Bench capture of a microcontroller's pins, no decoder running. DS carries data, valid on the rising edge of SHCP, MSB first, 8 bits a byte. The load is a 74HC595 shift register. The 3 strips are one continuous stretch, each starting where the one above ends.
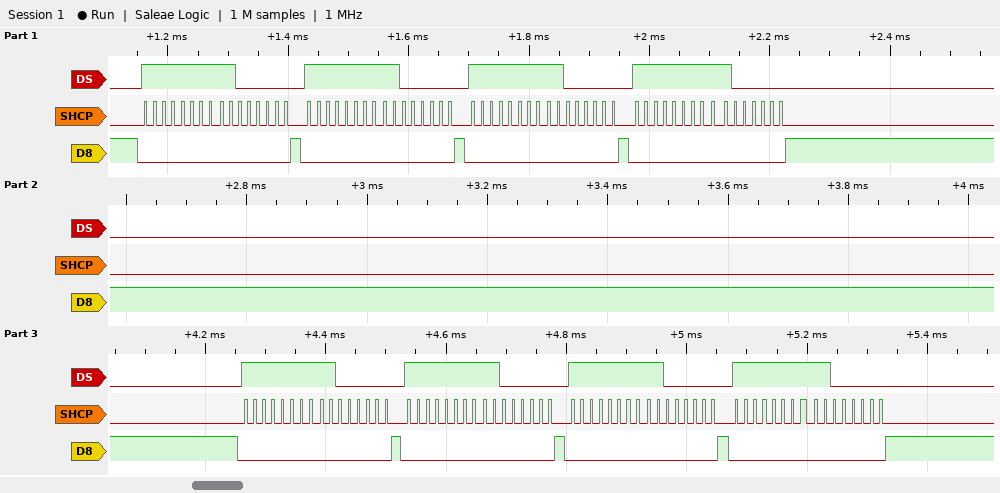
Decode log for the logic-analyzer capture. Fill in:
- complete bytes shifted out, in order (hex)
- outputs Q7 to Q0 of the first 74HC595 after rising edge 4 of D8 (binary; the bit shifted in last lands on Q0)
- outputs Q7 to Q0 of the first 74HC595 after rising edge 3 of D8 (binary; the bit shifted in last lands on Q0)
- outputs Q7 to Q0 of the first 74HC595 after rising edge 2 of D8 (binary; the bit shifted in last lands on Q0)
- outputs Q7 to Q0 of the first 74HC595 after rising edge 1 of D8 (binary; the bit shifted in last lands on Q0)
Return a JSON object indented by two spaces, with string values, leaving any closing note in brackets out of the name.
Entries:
{
  "complete bytes shifted out, in order": "0xFF 0xC0 0xFF 0xC0 0xFF 0xC0 0xFF 0xC0 0xFF 0xC0 0xFF 0xC0 0xFF 0xC0 0xFF 0xC0",
  "outputs Q7 to Q0 of the first 74HC595 after rising edge 4 of D8": "11000000",
  "outputs Q7 to Q0 of the first 74HC595 after rising edge 3 of D8": "11000000",
  "outputs Q7 to Q0 of the first 74HC595 after rising edge 2 of D8": "11000000",
  "outputs Q7 to Q0 of the first 74HC595 after rising edge 1 of D8": "11000000"
}
